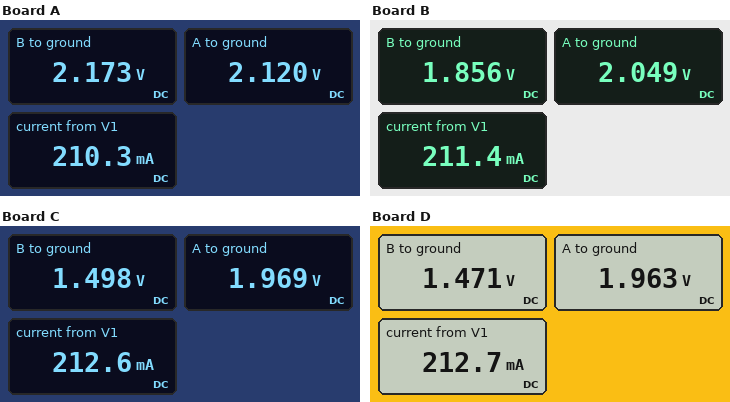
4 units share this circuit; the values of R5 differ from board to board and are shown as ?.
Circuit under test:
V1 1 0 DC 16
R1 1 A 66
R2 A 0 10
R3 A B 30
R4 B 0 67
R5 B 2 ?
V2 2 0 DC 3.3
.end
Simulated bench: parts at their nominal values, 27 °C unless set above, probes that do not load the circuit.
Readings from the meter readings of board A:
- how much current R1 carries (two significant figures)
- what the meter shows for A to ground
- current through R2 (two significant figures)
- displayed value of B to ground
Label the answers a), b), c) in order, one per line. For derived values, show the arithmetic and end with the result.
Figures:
a) (16 V - 2.12 V) / 66 Ω = 210 mA
b) 2.120 V
c) (2.12 V) / 10 Ω = 210 mA
d) 2.173 V
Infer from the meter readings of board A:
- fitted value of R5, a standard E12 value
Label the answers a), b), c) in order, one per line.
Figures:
a) 33 Ω
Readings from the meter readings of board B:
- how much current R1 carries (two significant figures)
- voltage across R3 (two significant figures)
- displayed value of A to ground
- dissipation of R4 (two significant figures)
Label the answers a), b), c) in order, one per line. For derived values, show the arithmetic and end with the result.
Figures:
a) (16 V - 2.049 V) / 66 Ω = 210 mA
b) 2.049 V - 1.856 V = 190 mV
c) 2.049 V
d) (1.856 V)^2 / 67 Ω = 51 mW
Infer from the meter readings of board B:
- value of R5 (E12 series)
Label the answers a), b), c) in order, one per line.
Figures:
a) 68 Ω
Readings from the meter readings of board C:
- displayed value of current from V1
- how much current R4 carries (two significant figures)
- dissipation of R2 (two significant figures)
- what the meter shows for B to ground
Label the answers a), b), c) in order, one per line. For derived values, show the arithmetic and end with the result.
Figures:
a) 212.6 mA
b) (1.498 V) / 67 Ω = 22 mA
c) (1.969 V)^2 / 10 Ω = 390 mW
d) 1.498 V
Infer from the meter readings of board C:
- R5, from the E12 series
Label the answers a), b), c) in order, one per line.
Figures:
a) 270 Ω
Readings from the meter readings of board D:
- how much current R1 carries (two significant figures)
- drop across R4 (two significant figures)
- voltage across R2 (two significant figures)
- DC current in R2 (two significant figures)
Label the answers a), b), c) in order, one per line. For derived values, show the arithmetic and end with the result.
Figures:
a) (16 V - 1.963 V) / 66 Ω = 210 mA
b) 1.471 V = 1.5 V
c) 1.963 V = 2.0 V
d) (1.963 V) / 10 Ω = 200 mA
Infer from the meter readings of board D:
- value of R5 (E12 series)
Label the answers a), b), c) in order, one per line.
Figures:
a) 330 Ω
